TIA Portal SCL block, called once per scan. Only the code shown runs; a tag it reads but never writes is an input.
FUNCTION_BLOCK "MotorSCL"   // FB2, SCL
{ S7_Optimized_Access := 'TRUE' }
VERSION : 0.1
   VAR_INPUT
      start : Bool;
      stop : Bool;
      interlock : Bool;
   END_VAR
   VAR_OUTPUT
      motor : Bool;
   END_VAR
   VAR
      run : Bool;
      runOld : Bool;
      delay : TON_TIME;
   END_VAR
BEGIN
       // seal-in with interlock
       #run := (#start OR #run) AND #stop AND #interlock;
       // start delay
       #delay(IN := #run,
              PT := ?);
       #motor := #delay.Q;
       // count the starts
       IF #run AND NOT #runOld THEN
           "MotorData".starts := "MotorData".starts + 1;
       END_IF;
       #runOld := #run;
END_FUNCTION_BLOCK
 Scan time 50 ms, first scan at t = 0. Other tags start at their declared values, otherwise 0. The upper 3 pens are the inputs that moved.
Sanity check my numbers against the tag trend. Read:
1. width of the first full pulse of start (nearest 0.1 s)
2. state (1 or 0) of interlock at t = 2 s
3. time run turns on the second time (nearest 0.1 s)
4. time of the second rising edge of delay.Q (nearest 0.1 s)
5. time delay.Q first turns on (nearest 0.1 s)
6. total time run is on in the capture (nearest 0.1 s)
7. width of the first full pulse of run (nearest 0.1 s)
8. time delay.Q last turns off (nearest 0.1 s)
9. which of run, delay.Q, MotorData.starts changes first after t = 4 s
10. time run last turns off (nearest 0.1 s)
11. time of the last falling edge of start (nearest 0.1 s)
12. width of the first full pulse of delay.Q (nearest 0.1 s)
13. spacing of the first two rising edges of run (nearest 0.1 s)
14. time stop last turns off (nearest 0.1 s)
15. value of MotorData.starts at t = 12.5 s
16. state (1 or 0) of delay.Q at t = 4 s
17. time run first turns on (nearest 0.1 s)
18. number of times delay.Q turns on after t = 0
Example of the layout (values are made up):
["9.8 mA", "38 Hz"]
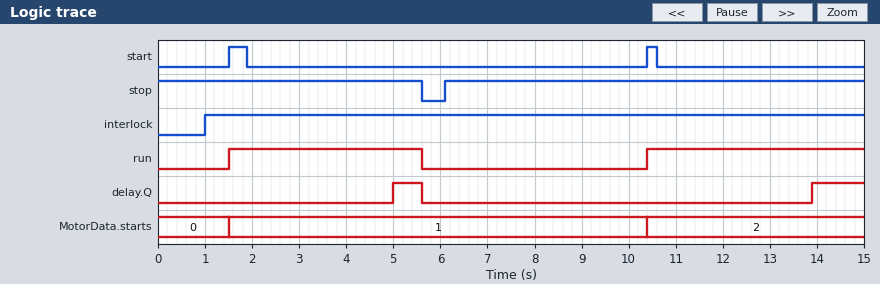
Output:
["0.4 s", "1", "10.4 s", "13.9 s", "5.0 s", "8.7 s", "4.1 s", "5.6 s", "delay.Q", "5.6 s", "10.6 s", "0.6 s", "8.9 s", "5.6 s", "2", "0", "1.5 s", "2"]
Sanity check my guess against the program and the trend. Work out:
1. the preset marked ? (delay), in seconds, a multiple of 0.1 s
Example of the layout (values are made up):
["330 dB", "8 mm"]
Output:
["3.5 s"]
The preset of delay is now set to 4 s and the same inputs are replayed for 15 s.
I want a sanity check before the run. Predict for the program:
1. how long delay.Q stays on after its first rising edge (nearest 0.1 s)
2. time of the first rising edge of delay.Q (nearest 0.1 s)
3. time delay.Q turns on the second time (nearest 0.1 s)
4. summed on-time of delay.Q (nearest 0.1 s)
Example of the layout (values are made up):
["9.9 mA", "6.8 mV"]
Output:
["0.1 s", "5.5 s", "14.4 s", "0.7 s"]
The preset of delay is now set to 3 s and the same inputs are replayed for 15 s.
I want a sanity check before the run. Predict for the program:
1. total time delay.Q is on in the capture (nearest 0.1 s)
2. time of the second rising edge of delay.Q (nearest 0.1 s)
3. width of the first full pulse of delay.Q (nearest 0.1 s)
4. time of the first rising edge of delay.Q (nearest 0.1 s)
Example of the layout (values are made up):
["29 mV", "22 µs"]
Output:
["2.7 s", "13.4 s", "1.1 s", "4.5 s"]
